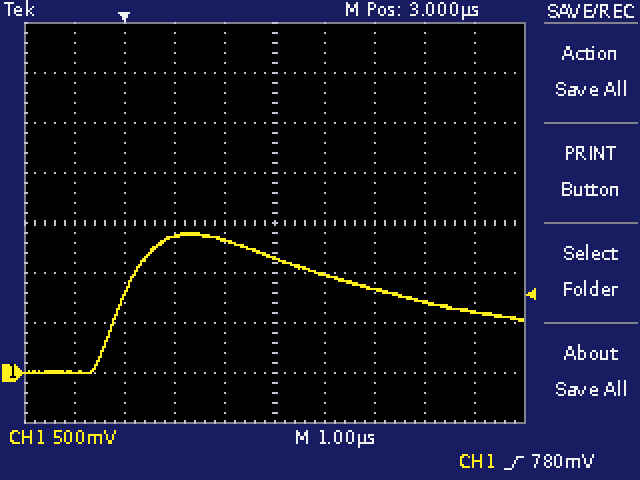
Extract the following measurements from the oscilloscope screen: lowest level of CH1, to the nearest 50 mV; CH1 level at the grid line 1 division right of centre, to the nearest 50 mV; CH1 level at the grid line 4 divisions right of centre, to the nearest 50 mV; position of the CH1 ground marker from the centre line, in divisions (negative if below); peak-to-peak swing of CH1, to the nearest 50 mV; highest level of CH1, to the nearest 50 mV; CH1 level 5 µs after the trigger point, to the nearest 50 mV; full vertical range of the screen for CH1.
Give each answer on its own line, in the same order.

0 mV
1.00 V
600 mV
-3.0 div
1.40 V
1.40 V
850 mV
4 V
